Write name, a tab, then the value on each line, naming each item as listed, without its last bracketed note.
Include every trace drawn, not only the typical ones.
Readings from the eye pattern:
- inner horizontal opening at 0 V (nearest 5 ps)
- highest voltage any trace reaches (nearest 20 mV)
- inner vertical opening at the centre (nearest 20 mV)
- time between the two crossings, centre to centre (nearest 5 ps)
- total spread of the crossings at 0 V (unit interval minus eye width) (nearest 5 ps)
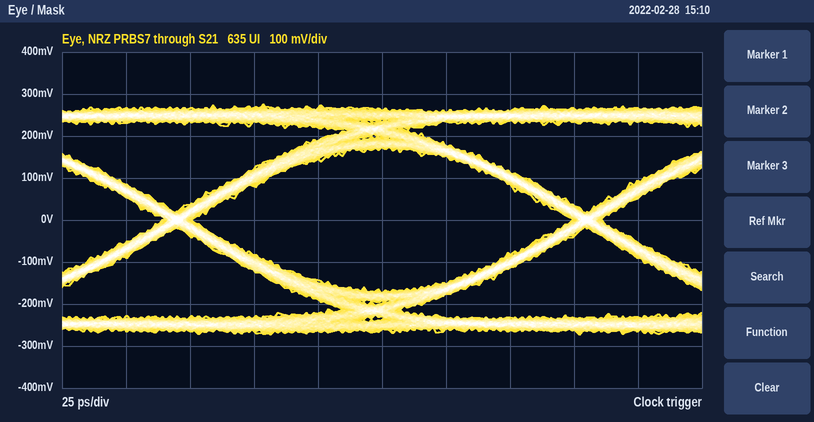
inner horizontal opening at 0 V	150 ps
highest voltage any trace reaches	280 mV
inner vertical opening at the centre	340 mV
time between the two crossings, centre to centre	160 ps
total spread of the crossings at 0 V (unit interval minus eye width)	10 ps
